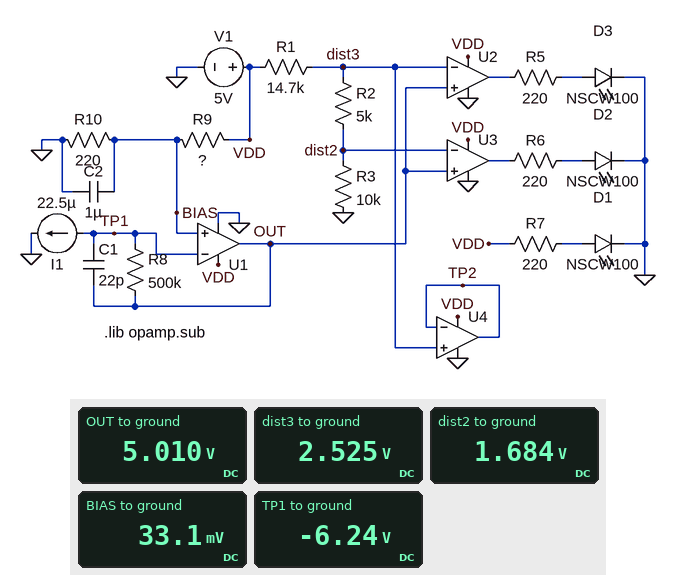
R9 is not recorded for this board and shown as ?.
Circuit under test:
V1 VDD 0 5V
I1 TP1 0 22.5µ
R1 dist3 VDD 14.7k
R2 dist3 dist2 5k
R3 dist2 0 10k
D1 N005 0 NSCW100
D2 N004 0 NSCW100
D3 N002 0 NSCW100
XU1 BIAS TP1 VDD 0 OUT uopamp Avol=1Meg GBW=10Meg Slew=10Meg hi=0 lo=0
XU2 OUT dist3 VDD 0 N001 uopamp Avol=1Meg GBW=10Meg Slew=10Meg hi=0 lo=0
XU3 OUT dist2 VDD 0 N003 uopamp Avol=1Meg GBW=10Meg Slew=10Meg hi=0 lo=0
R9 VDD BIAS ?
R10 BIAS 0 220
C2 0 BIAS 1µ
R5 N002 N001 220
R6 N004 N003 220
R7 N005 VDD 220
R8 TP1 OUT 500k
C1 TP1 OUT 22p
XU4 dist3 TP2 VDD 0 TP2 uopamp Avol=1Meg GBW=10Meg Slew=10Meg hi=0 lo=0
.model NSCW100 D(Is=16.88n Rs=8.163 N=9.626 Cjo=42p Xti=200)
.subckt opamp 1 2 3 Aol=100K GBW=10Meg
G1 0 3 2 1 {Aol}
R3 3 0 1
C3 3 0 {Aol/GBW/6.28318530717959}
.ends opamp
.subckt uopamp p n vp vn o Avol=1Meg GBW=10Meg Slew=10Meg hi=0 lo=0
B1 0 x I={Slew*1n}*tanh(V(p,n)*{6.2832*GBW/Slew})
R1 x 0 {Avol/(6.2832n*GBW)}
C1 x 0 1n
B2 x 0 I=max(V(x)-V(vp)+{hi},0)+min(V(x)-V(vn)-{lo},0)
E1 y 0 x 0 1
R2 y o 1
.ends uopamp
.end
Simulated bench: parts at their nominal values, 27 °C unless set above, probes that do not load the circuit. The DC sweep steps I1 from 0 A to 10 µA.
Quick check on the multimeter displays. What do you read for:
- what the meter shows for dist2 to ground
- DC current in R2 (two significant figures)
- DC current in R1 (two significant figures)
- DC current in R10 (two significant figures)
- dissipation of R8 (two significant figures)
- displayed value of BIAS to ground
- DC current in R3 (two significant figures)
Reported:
1.684 V
170 µA
170 µA
150 µA
250 µW
33.1 mV
170 µA
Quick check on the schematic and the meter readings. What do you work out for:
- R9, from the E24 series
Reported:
33 kΩ
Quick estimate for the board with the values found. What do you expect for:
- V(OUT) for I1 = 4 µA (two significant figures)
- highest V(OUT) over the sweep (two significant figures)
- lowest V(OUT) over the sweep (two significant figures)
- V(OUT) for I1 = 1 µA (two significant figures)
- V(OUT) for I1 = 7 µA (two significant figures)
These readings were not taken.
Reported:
2.0 V
5.0 V
33 mV
530 mV
3.5 V
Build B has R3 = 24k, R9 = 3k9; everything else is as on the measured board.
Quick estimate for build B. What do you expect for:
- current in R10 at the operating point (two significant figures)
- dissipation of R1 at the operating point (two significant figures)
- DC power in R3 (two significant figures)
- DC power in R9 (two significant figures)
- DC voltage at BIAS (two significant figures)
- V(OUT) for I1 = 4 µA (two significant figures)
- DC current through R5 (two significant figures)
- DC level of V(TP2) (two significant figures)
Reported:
1.2 mA
190 µW
310 µW
5.7 mW
270 mV
2.3 V
7.7 mA
3.3 V
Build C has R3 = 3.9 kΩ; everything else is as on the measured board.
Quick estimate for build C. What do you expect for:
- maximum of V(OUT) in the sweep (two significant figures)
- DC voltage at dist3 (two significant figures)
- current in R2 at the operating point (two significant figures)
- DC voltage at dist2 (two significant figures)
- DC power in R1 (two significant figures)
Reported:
5.0 V
1.9 V
210 µA
830 mV
660 µW
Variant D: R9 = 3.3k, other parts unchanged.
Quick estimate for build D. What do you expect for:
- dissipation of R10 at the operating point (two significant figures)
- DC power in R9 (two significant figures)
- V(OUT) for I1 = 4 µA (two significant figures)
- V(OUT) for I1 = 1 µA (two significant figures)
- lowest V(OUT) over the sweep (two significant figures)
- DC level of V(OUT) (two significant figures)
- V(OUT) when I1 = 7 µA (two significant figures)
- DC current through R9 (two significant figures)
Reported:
440 µW
6.7 mW
2.3 V
810 mV
310 mV
5.0 V
3.8 V
1.4 mA
